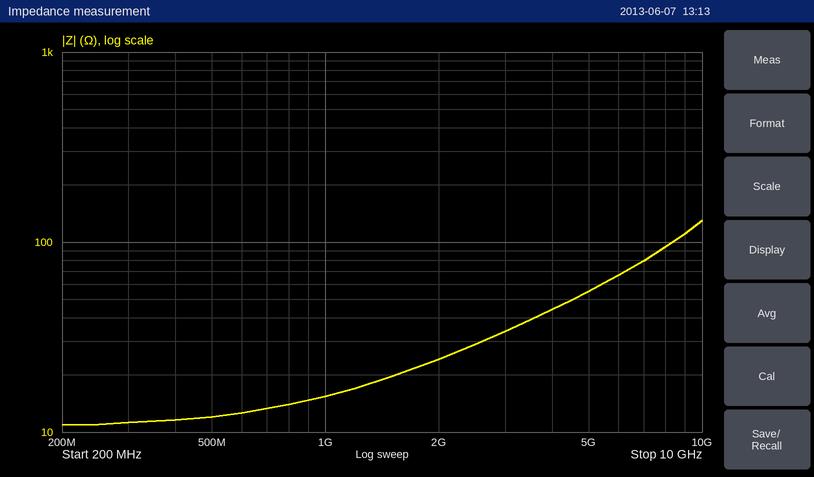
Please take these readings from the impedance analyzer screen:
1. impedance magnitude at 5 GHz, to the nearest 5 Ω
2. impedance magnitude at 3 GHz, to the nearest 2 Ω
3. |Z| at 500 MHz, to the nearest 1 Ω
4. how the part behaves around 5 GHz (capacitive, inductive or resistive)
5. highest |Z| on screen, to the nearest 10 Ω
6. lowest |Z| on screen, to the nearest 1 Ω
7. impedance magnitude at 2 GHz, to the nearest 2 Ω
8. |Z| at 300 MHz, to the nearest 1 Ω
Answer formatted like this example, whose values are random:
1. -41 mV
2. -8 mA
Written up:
1. 55 Ω
2. 34 Ω
3. 12 Ω
4. inductive
5. 130 Ω
6. 11 Ω
7. 24 Ω
8. 11 Ω
